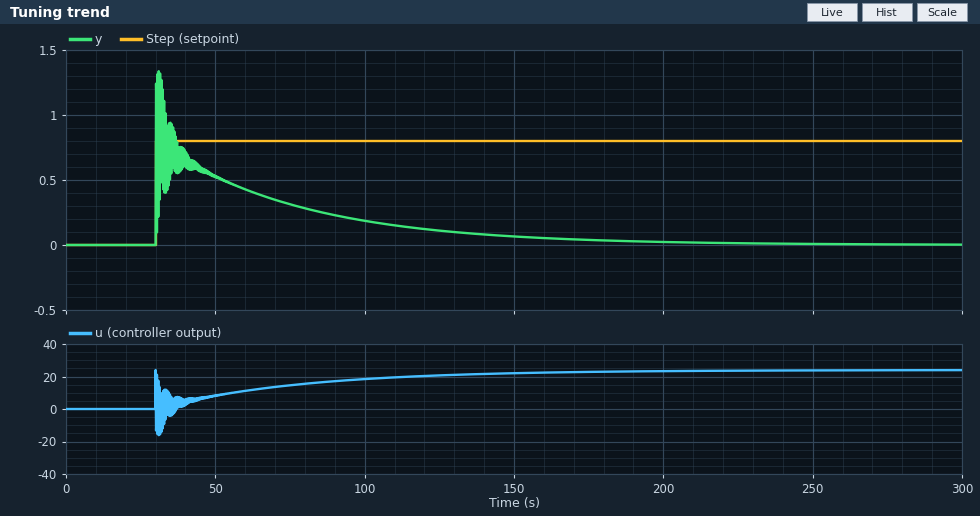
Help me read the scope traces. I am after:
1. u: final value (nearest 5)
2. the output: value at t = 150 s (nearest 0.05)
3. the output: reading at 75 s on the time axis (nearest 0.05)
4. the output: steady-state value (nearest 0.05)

25
0.05
0.30
0.00
